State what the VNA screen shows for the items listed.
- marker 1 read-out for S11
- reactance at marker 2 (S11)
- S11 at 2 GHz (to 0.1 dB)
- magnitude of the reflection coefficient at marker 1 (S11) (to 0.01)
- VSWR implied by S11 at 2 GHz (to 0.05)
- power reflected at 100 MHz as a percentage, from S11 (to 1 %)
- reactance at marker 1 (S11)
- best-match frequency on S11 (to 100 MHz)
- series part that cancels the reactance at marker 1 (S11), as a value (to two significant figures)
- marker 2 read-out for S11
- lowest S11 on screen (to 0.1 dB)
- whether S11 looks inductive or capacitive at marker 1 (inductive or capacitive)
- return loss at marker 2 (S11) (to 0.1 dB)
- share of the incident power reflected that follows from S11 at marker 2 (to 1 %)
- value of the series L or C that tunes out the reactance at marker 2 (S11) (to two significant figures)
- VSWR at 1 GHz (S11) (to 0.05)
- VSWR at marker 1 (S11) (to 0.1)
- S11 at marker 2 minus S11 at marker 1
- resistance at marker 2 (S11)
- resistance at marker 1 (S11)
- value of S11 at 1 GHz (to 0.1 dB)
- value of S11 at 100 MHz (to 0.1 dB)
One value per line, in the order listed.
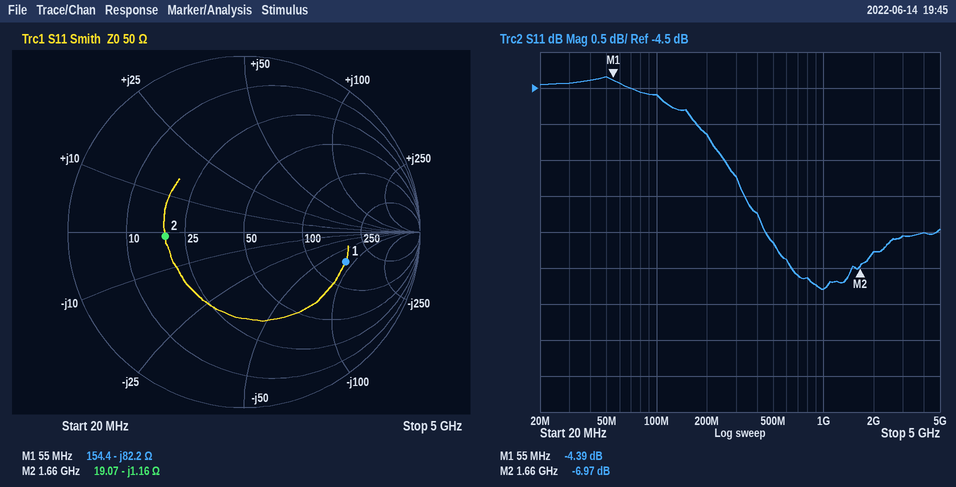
-4.39 dB
-1.16 Ω
-6.8 dB
0.60
2.70
35 %
-82.2 Ω
1.0 GHz
240 nH
-6.97 dB
-7.3 dB
capacitive
7.0 dB
20 %
110 pH
2.50
4.0
-2.58 dB
19.07 Ω
154.4 Ω
-7.3 dB
-4.6 dB
